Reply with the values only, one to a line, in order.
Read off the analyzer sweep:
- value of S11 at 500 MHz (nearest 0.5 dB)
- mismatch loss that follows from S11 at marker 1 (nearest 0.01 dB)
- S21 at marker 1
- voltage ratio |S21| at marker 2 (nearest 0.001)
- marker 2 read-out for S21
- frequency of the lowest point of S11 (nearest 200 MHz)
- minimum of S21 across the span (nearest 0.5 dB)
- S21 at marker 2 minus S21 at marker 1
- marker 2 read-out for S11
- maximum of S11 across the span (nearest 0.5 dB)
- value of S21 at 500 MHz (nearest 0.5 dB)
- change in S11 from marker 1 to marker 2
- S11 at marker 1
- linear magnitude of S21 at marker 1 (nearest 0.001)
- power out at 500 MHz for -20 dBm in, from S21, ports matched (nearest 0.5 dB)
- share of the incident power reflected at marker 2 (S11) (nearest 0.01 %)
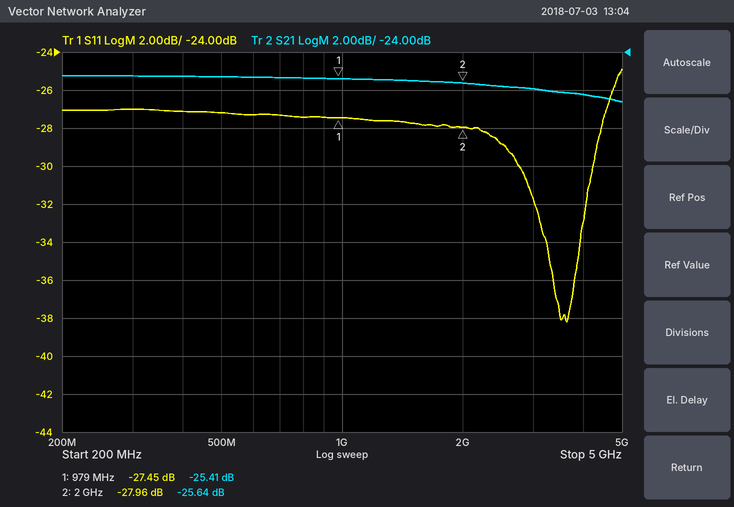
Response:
-27.0 dB
0.01 dB
-25.41 dB
0.052
-25.64 dB
3.6 GHz
-26.5 dB
-0.23 dB
-27.96 dB
-25.0 dB
-25.5 dB
-0.51 dB
-27.45 dB
0.054
-45.5 dBm
0.16 %
